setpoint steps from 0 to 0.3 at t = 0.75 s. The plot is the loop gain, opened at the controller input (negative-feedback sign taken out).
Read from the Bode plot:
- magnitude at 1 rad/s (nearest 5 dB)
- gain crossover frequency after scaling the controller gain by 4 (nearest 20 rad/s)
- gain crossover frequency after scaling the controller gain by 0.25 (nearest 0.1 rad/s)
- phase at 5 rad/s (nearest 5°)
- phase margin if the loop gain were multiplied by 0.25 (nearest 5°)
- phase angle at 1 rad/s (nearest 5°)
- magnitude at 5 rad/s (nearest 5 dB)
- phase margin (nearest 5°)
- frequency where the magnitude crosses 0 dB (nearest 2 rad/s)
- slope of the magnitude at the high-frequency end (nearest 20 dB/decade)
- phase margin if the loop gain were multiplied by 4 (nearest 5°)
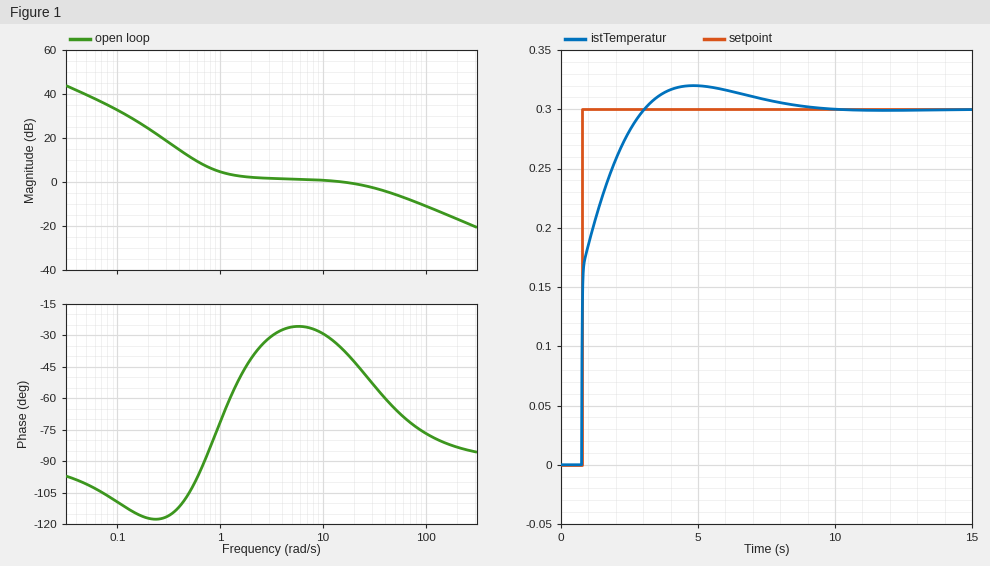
5 dB
120 rad/s
0.5 rad/s
-25°
75°
-70°
0 dB
145°
16 rad/s
-20 dB/decade
100°
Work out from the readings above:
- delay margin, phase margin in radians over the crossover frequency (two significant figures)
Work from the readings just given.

0.16 s
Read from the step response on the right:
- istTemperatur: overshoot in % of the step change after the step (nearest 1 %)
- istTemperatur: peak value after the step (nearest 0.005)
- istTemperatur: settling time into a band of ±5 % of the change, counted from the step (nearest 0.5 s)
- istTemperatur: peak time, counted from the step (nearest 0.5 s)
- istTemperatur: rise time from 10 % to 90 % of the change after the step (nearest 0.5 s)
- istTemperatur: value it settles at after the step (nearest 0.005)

7 %
0.320
5.5 s
4.0 s
1.5 s
0.300
